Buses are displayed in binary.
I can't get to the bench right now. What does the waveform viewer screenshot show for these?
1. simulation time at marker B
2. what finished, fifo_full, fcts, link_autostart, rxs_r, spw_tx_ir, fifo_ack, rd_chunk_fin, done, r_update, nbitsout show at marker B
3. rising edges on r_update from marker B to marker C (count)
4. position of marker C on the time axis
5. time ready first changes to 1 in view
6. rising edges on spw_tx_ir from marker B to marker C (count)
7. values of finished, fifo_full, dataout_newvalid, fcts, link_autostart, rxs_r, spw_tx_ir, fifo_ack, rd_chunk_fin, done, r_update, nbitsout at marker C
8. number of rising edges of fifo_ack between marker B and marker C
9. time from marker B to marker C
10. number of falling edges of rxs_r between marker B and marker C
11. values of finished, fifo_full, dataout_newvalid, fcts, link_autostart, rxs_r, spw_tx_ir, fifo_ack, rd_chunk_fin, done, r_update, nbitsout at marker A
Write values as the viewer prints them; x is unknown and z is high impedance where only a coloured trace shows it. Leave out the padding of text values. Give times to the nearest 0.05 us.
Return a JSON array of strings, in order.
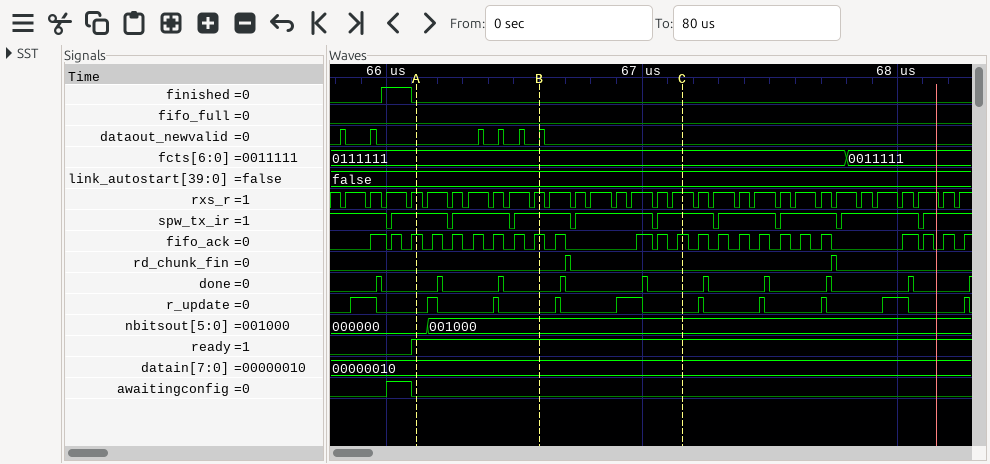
["66.6 us", "finished=0, fifo_full=0, fcts=0111111, link_autostart=false, rxs_r=1, spw_tx_ir=1, fifo_ack=1, rd_chunk_fin=0, done=0, r_update=0, nbitsout=001000", "2", "67.15 us", "66.1 us", "2", "finished=0, fifo_full=0, dataout_newvalid=0, fcts=0111111, link_autostart=false, rxs_r=1, spw_tx_ir=1, fifo_ack=1, rd_chunk_fin=0, done=0, r_update=0, nbitsout=001000", "4", "0.55 us", "7", "finished=0, fifo_full=0, dataout_newvalid=0, fcts=0111111, link_autostart=false, rxs_r=1, spw_tx_ir=1, fifo_ack=1, rd_chunk_fin=0, done=0, r_update=0, nbitsout=000000"]
